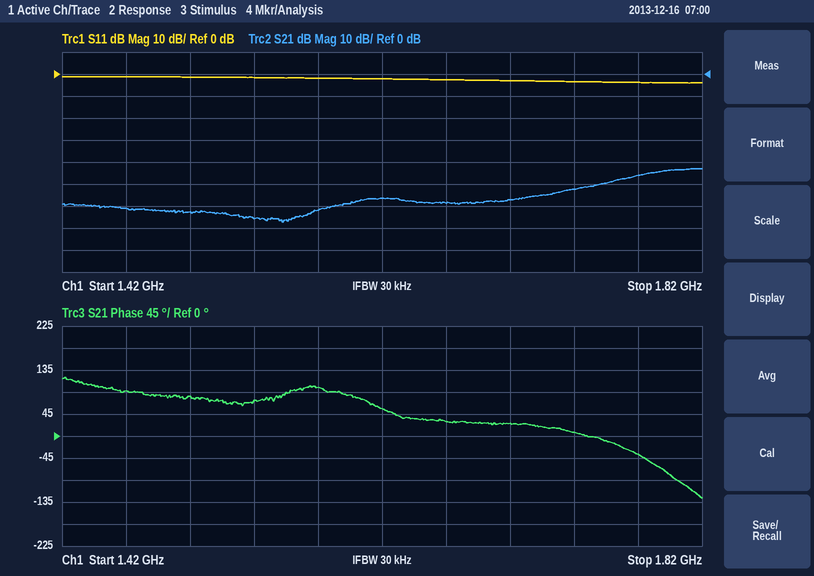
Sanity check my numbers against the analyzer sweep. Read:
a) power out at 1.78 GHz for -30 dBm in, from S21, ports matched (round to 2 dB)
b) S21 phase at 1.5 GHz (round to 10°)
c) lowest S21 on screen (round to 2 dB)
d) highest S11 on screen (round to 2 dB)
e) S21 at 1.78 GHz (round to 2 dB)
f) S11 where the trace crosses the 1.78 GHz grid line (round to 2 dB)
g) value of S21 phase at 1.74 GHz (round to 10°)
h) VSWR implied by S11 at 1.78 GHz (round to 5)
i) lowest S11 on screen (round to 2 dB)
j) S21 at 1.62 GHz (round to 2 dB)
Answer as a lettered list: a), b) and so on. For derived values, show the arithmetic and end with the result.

a) -30 dBm + (-46 dB) = -76 dBm
b) 80°
c) -68 dB
d) -2 dB
e) -46 dB
f) -4 dB
g) 10°
h) |Γ| = 10^(-4/20) = 0.6310; VSWR = (1 + 0.6310)/(1 − 0.6310) ≈ 4.42, so 5 to the nearest 5
i) -4 dB
j) -56 dB
